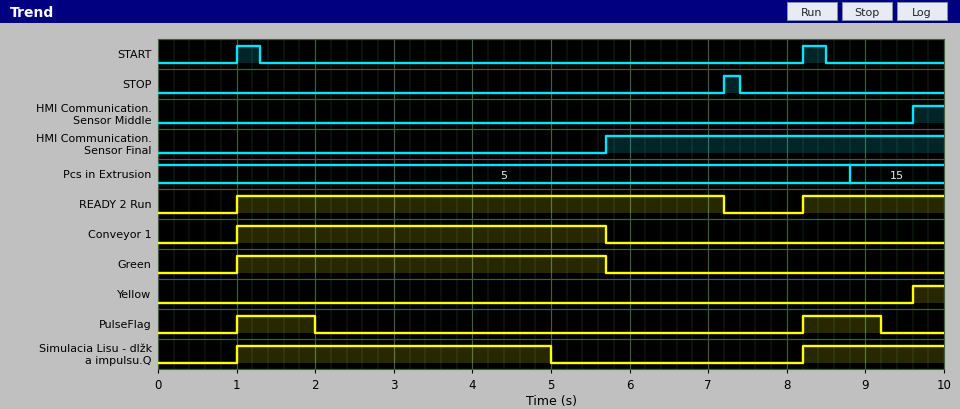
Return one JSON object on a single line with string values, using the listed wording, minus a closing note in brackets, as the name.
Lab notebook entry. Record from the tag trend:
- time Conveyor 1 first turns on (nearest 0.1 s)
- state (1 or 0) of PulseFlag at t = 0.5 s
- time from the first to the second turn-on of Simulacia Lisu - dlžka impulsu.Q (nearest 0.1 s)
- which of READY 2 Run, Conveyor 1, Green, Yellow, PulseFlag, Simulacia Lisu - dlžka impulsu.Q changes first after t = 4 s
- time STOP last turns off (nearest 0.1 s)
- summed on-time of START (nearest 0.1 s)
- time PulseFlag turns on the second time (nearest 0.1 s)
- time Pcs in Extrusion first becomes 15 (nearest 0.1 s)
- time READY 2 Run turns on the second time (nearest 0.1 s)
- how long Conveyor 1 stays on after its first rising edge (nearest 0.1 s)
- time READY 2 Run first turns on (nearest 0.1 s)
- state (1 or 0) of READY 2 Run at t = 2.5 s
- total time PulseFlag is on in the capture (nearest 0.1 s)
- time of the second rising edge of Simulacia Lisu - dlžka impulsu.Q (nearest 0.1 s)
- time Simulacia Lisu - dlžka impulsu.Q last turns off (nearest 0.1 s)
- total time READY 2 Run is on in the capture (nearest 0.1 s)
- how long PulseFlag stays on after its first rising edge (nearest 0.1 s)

{"time Conveyor 1 first turns on": "1.0 s", "state (1 or 0) of PulseFlag at t = 0.5 s": "0", "time from the first to the second turn-on of Simulacia Lisu - dlžka impulsu.Q": "7.2 s", "which of READY 2 Run, Conveyor 1, Green, Yellow, PulseFlag, Simulacia Lisu - dlžka impulsu.Q changes first after t = 4 s": "Simulacia Lisu - dlžka impulsu.Q", "time STOP last turns off": "7.4 s", "summed on-time of START": "0.6 s", "time PulseFlag turns on the second time": "8.2 s", "time Pcs in Extrusion first becomes 15": "8.8 s", "time READY 2 Run turns on the second time": "8.2 s", "how long Conveyor 1 stays on after its first rising edge": "4.7 s", "time READY 2 Run first turns on": "1.0 s", "state (1 or 0) of READY 2 Run at t = 2.5 s": "1", "total time PulseFlag is on in the capture": "2.0 s", "time of the second rising edge of Simulacia Lisu - dlžka impulsu.Q": "8.2 s", "time Simulacia Lisu - dlžka impulsu.Q last turns off": "5.0 s", "total time READY 2 Run is on in the capture": "8.0 s", "how long PulseFlag stays on after its first rising edge": "1.0 s"}
